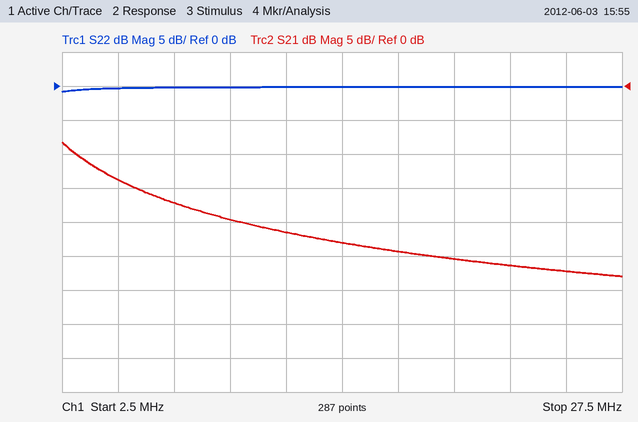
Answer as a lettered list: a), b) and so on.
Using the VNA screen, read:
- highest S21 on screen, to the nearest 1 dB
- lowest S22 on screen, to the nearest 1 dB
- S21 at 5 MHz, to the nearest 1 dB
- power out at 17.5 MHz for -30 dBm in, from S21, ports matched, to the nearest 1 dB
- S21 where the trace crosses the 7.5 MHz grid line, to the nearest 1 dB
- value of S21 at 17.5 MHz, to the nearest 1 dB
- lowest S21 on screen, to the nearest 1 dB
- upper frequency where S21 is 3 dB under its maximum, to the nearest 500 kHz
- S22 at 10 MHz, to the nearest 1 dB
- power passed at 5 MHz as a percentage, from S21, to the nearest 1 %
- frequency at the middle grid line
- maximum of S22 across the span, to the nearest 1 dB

a) -8 dB
b) -1 dB
c) -14 dB
d) -54 dBm
e) -17 dB
f) -24 dB
g) -28 dB
h) 3.5 MHz
i) 0 dB
j) 4 %
k) 15 MHz
l) 0 dB
